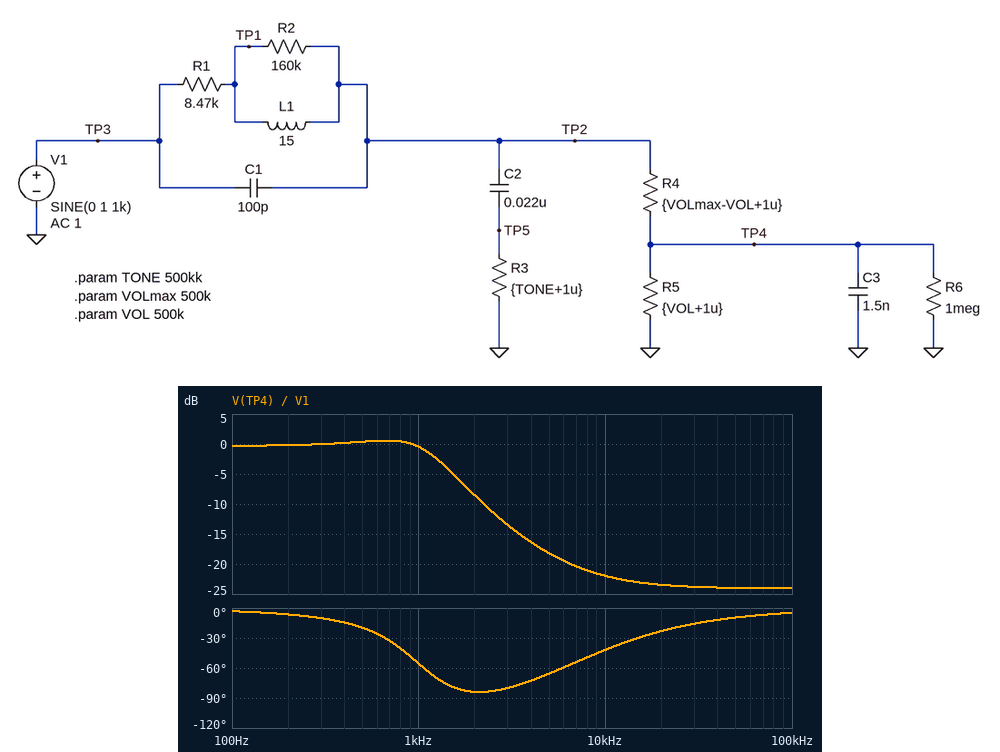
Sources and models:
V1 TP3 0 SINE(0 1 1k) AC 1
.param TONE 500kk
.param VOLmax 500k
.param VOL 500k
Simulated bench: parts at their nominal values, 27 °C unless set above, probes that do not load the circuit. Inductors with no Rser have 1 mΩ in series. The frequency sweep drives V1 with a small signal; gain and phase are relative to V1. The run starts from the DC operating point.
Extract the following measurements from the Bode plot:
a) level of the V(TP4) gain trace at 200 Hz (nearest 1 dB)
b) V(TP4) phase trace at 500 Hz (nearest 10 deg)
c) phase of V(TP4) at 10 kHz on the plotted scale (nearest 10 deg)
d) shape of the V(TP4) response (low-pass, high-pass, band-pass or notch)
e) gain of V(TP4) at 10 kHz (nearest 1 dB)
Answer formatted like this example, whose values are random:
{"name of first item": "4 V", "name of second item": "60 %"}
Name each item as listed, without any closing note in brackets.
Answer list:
{"level of the V(TP4) gain trace at 200 Hz": "0 dB", "V(TP4) phase trace at 500 Hz": "-20 deg", "phase of V(TP4) at 10 kHz on the plotted scale": "-40 deg", "shape of the V(TP4) response": "low-pass", "gain of V(TP4) at 10 kHz": "-22 dB"}
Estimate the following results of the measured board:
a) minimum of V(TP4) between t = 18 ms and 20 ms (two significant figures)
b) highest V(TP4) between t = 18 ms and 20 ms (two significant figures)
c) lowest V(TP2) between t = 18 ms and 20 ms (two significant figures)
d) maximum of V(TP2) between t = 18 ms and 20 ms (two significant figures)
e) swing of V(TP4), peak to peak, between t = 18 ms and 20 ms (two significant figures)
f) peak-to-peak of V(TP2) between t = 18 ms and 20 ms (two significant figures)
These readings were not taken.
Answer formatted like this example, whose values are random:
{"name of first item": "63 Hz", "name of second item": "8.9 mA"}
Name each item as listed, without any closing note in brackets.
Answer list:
{"minimum of V(TP4) between t = 18 ms and 20 ms": "-950 mV", "highest V(TP4) between t = 18 ms and 20 ms": "950 mV", "lowest V(TP2) between t = 18 ms and 20 ms": "-950 mV", "maximum of V(TP2) between t = 18 ms and 20 ms": "950 mV", "swing of V(TP4), peak to peak, between t = 18 ms and 20 ms": "1.9 V", "peak-to-peak of V(TP2) between t = 18 ms and 20 ms": "1.9 V"}
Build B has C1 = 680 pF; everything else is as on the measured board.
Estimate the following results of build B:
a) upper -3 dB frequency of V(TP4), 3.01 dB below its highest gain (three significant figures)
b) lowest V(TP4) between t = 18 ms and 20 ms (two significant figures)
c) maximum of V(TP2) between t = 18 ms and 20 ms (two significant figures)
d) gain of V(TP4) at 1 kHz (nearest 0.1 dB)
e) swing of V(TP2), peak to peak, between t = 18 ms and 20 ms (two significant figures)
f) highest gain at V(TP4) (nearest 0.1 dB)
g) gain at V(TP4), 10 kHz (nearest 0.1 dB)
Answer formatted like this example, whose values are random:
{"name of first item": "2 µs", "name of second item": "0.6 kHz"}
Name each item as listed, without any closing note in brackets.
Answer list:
{"upper -3 dB frequency of V(TP4), 3.01 dB below its highest gain": "962 Hz", "lowest V(TP4) between t = 18 ms and 20 ms": "-680 mV", "maximum of V(TP2) between t = 18 ms and 20 ms": "680 mV", "gain of V(TP4) at 1 kHz": "-3.3 dB", "swing of V(TP2), peak to peak, between t = 18 ms and 20 ms": "1.4 V", "highest gain at V(TP4)": "0.2 dB", "gain at V(TP4), 10 kHz": "-10.2 dB"}
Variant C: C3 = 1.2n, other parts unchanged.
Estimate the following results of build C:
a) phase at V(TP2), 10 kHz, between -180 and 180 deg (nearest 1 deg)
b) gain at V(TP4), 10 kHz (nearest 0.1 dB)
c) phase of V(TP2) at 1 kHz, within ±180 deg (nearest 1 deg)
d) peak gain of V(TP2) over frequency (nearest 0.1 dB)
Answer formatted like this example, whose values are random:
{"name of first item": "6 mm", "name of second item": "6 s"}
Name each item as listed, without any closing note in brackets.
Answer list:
{"phase at V(TP2), 10 kHz, between -180 and 180 deg": "-40 deg", "gain at V(TP4), 10 kHz": "-20.2 dB", "phase of V(TP2) at 1 kHz, within ±180 deg": "-46 deg", "peak gain of V(TP2) over frequency": "0.2 dB"}
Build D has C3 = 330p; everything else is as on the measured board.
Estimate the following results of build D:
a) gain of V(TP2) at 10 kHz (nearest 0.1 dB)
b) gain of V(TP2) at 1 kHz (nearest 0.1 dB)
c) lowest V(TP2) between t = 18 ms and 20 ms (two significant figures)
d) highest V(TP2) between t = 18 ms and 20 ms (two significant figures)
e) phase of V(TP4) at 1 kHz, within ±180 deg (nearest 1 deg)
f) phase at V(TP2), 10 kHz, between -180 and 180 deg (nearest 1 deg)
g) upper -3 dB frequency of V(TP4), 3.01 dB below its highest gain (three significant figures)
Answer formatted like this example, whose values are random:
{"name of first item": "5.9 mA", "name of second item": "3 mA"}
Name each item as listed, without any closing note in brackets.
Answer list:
{"gain of V(TP2) at 10 kHz": "-11.0 dB", "gain of V(TP2) at 1 kHz": "-1.7 dB", "lowest V(TP2) between t = 18 ms and 20 ms": "-820 mV", "highest V(TP2) between t = 18 ms and 20 ms": "820 mV", "phase of V(TP4) at 1 kHz, within ±180 deg": "-23 deg", "phase at V(TP2), 10 kHz, between -180 and 180 deg": "-25 deg", "upper -3 dB frequency of V(TP4), 3.01 dB below its highest gain": "1.67 kHz"}
